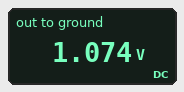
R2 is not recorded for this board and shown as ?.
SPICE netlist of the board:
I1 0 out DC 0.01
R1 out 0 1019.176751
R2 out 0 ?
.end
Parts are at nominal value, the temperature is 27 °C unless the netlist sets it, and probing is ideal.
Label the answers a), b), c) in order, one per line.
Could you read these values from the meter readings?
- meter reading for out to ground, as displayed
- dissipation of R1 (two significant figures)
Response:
a) 1.074 V
b) 1.1 mW
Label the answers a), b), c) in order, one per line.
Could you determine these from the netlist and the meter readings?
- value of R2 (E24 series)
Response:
a) 120 Ω
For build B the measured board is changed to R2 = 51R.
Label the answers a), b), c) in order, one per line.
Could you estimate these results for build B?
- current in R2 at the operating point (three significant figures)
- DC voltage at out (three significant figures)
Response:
a) 9.52 mA
b) 486 mV
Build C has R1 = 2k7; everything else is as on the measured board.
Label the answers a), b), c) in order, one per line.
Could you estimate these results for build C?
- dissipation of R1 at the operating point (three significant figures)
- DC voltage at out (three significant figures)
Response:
a) 489 µW
b) 1.15 V
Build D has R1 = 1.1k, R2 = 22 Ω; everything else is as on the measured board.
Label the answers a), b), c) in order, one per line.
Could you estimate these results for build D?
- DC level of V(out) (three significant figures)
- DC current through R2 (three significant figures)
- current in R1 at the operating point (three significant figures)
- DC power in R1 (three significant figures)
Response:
a) 216 mV
b) 9.80 mA
c) 196 µA
d) 42.3 µW
